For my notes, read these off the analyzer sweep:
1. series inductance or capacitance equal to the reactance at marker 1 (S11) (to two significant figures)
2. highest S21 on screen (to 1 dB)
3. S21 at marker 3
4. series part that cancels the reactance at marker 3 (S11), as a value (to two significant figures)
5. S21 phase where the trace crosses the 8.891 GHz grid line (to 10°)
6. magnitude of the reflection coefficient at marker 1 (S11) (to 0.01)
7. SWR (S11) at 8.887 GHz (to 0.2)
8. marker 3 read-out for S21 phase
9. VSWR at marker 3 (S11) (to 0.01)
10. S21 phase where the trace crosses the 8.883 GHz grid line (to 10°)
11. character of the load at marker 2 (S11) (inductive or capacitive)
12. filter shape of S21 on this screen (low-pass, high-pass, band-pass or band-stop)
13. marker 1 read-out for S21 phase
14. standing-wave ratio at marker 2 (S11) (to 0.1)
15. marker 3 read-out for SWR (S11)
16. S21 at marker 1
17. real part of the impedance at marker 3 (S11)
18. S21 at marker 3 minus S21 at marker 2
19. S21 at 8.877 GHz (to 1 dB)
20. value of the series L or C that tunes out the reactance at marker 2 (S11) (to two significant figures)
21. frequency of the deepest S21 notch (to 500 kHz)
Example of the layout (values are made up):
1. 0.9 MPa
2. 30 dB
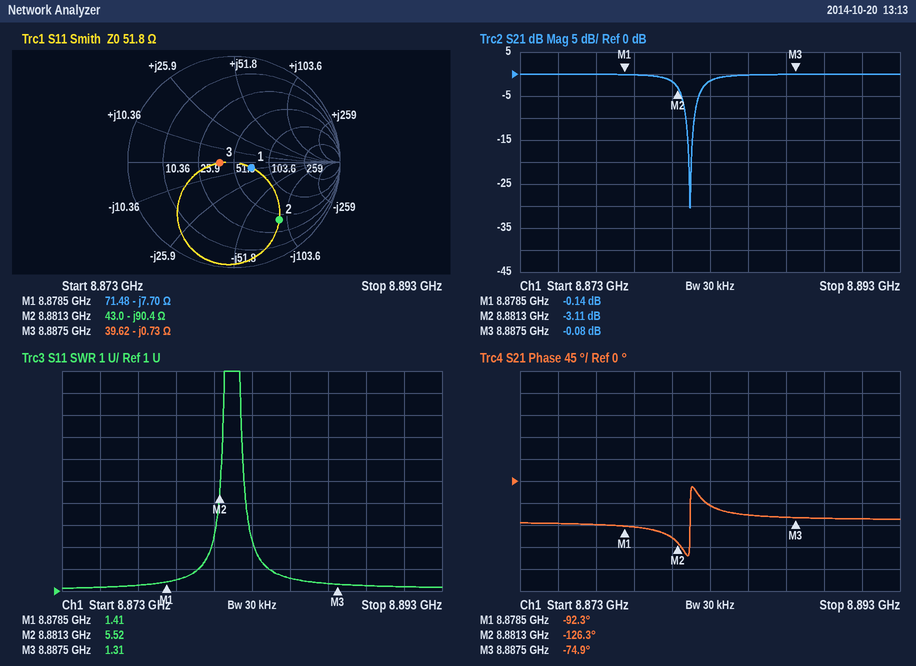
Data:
1. 2.3 pF
2. 0 dB
3. -0.08 dB
4. 13 pH
5. -80°
6. 0.17
7. 1.4
8. -74.9°
9. 1.31
10. -50°
11. capacitive
12. band-stop
13. -92.3°
14. 5.5
15. 1.31
16. -0.14 dB
17. 39.62 Ω
18. 3.03 dB
19. 0 dB
20. 1.6 nH
21. 8.8820 GHz
